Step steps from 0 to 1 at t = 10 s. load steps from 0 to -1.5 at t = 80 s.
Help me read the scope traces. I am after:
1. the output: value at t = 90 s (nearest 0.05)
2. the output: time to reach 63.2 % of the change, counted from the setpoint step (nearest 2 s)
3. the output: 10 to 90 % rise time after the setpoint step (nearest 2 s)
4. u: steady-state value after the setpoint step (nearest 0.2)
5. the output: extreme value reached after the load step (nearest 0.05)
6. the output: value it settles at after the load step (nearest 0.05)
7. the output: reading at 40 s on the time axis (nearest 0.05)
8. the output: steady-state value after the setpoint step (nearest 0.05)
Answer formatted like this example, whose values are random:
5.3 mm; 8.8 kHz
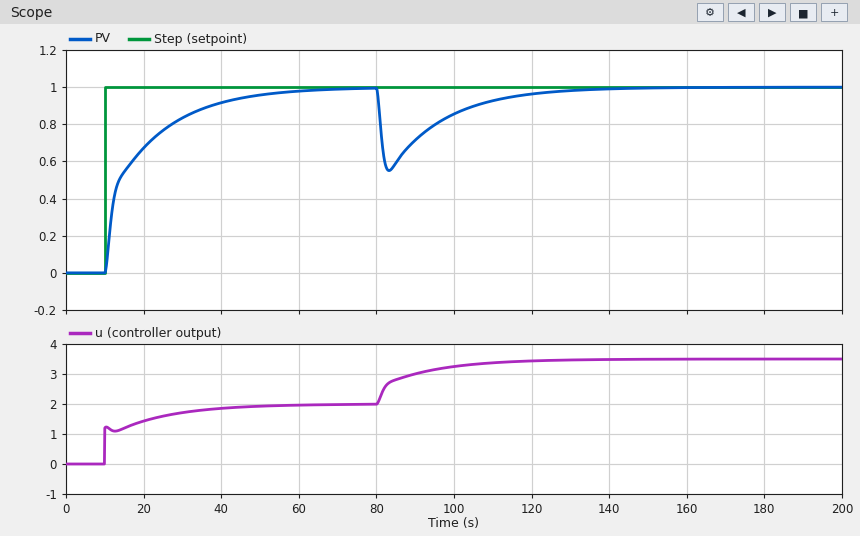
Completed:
0.70; 8 s; 26 s; 2.0; 0.55; 1.00; 0.90; 1.00
